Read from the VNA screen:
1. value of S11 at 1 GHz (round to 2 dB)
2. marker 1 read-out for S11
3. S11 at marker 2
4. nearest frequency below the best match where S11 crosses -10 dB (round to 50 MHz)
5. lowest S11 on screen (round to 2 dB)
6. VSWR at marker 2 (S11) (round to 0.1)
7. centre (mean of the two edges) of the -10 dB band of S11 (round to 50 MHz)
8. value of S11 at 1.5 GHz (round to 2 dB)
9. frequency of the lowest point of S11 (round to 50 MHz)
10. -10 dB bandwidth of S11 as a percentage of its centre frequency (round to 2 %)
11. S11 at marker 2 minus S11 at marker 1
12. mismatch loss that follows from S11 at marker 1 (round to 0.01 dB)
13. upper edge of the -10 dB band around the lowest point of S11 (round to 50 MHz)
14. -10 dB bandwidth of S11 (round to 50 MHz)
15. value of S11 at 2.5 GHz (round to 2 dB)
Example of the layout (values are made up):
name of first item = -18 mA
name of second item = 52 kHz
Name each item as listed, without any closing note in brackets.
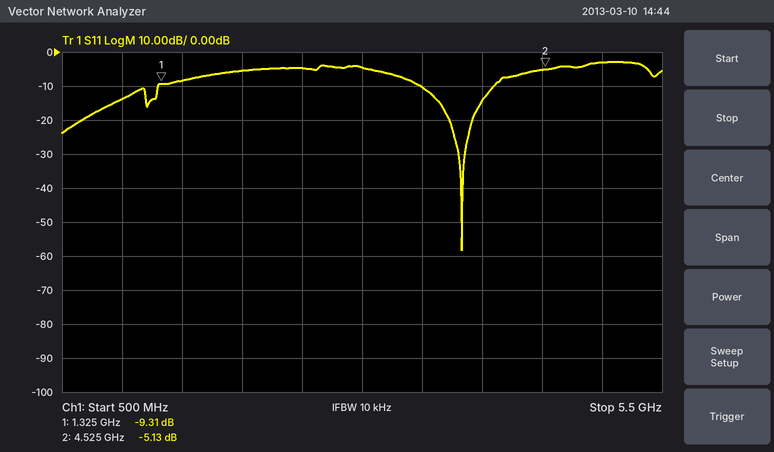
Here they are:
value of S11 at 1 GHz = -14 dB
marker 1 read-out for S11 = -9.31 dB
S11 at marker 2 = -5.13 dB
nearest frequency below the best match where S11 crosses -10 dB = 3.50 GHz
lowest S11 on screen = -58 dB
VSWR at marker 2 (S11) = 3.5
centre (mean of the two edges) of the -10 dB band of S11 = 3.80 GHz
value of S11 at 1.5 GHz = -8 dB
frequency of the lowest point of S11 = 3.85 GHz
-10 dB bandwidth of S11 as a percentage of its centre frequency = 16 %
S11 at marker 2 minus S11 at marker 1 = 4.18 dB
mismatch loss that follows from S11 at marker 1 = 0.54 dB
upper edge of the -10 dB band around the lowest point of S11 = 4.10 GHz
-10 dB bandwidth of S11 = 600 MHz
value of S11 at 2.5 GHz = -4 dB
